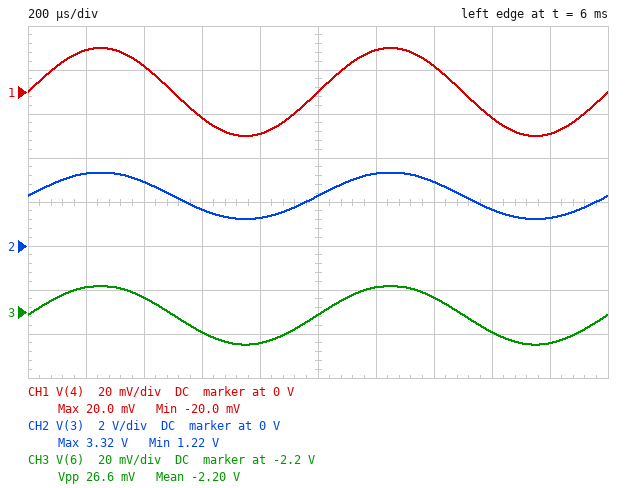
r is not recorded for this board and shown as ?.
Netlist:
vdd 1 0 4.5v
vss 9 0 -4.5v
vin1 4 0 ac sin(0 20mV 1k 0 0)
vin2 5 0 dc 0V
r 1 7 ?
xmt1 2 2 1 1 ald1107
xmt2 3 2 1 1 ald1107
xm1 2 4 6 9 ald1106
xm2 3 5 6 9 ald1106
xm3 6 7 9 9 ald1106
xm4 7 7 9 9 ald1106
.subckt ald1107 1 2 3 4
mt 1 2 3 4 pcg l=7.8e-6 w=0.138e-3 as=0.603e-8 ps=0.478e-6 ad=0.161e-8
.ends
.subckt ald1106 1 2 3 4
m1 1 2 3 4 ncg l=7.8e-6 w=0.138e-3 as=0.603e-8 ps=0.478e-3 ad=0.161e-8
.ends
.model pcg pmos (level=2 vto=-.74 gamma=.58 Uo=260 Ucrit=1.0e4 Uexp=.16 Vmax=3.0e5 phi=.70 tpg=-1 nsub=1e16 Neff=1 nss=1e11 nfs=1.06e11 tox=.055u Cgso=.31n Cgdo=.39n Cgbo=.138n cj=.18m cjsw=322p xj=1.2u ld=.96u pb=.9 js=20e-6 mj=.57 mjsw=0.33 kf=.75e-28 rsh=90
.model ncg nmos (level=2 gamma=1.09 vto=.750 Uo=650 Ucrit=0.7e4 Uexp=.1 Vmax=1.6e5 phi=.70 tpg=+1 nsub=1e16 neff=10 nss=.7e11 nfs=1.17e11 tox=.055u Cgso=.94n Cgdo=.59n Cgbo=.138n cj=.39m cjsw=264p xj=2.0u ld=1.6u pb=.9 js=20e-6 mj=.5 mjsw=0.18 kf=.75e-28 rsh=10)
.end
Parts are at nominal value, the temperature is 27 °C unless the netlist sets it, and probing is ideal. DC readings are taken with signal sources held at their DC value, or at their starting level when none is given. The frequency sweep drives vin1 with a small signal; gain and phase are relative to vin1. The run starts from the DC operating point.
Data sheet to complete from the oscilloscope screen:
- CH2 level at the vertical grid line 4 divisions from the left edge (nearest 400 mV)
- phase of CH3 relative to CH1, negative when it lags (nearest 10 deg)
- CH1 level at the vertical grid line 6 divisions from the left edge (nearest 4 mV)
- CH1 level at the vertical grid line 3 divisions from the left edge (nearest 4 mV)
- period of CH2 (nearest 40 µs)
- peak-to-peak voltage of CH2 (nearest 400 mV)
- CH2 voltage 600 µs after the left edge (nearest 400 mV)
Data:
1.2 V
0 deg
20 mV
-12 mV
1.00 ms
2.0 V
1.6 V
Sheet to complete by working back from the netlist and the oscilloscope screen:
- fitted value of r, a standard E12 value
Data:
15 kΩ
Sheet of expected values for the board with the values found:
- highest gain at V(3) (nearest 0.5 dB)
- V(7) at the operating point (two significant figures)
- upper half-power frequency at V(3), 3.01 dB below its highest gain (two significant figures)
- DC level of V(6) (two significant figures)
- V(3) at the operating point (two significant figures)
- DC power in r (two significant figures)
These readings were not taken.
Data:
34.5 dB
-2.6 V
3.4 MHz
-2.2 V
2.3 V
3.4 mW
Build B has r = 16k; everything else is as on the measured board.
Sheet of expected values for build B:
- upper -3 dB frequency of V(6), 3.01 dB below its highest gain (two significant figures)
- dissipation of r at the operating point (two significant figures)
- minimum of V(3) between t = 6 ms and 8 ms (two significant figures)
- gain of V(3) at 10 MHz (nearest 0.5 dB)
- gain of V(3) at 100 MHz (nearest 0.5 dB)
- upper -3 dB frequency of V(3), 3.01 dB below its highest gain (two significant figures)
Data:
5.3 MHz
3.2 mW
1.3 V
24.0 dB
-0.5 dB
3.2 MHz
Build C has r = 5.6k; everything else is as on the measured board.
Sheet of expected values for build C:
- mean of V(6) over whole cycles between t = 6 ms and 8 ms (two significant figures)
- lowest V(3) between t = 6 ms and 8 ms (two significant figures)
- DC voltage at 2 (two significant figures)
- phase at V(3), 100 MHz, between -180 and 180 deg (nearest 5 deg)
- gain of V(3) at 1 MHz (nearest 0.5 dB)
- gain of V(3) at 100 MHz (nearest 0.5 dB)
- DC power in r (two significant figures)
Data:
-2.6 V
530 mV
1.4 V
-130 deg
32.5 dB
5.5 dB
7.4 mW
